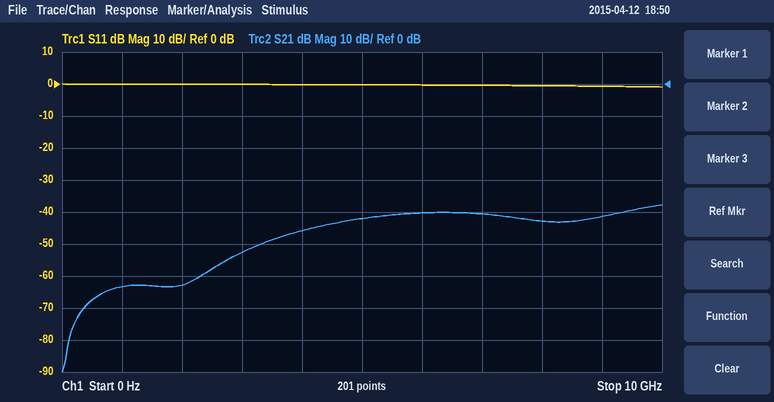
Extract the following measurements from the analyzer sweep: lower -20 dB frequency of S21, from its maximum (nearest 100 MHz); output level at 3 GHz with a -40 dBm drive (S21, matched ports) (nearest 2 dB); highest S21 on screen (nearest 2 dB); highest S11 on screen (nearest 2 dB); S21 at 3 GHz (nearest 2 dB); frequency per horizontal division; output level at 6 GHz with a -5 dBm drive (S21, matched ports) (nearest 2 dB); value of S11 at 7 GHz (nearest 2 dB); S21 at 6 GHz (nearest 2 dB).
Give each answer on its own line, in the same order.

2.5 GHz
-92 dBm
-38 dB
0 dB
-52 dB
1 GHz
-46 dBm
0 dB
-40 dB
